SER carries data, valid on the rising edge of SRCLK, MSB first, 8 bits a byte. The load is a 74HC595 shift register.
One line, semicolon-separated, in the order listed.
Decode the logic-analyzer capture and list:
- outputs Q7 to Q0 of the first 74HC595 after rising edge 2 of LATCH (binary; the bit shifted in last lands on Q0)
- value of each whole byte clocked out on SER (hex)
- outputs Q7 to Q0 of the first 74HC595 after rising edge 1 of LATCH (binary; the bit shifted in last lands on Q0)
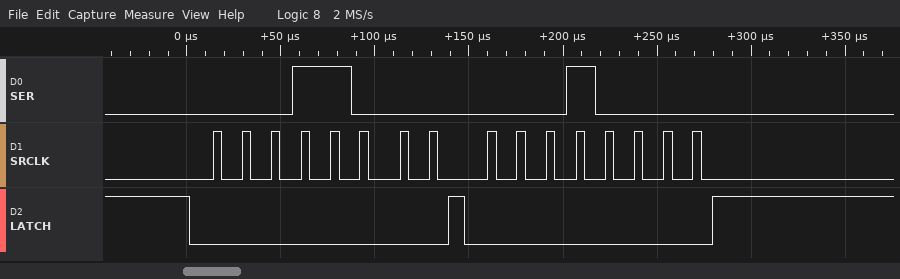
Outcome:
00010000; 18 10; 00011000
